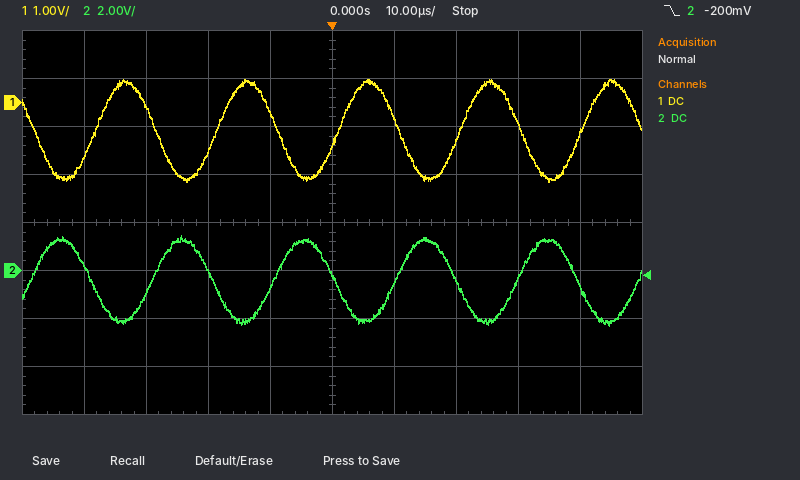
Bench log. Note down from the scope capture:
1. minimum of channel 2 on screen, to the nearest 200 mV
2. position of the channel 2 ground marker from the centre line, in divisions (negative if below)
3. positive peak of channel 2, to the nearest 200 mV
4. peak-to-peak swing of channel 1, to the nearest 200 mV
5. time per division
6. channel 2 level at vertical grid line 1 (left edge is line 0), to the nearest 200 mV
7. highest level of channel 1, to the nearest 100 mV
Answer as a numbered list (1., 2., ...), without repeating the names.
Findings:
1. -2.2 V
2. -1.0 div
3. 1.4 V
4. 2.2 V
5. 10 µs
6. 200 mV
7. 500 mV
